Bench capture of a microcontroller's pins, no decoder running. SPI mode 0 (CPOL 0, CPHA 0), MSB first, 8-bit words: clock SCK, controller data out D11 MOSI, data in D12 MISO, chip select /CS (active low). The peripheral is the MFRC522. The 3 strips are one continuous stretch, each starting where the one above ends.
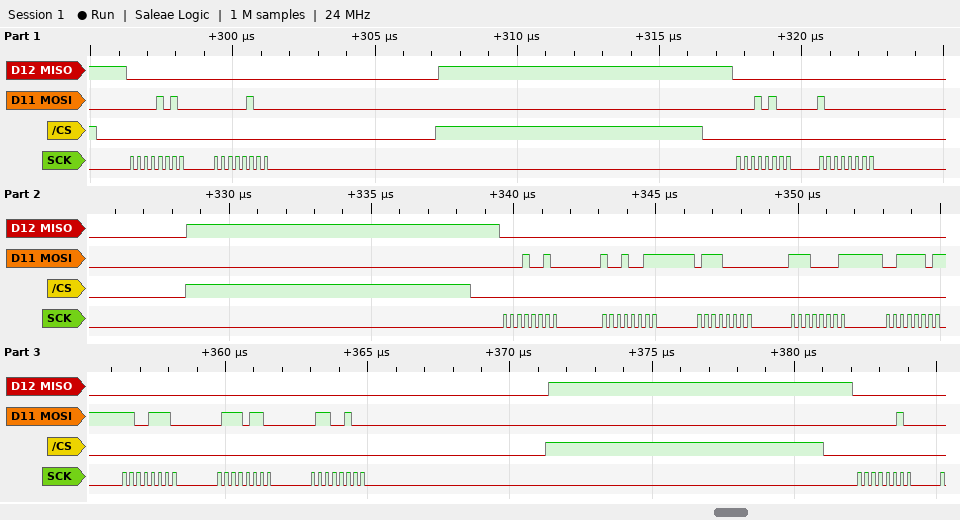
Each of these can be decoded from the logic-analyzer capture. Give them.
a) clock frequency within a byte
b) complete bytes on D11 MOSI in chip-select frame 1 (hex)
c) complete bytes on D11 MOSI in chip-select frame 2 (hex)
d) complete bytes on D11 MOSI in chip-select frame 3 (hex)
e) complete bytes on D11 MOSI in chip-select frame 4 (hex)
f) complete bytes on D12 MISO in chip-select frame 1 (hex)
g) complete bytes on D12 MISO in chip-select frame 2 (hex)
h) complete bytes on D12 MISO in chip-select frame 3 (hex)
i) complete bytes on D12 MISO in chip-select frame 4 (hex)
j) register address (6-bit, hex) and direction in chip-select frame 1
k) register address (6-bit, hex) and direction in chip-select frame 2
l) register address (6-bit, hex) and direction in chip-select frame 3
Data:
4 MHz
0x0A 0x04
0x14 0x80
0x12 0x93 0x70 0xE1 0x3D 0xCE 0x76 0x64
0x02
0x00 0x00
0x00 0x00
0x00 0x00 0x00 0x00 0x00 0x00 0x00 0x00
0x00
0x05 write
0x0A write
0x09 write
